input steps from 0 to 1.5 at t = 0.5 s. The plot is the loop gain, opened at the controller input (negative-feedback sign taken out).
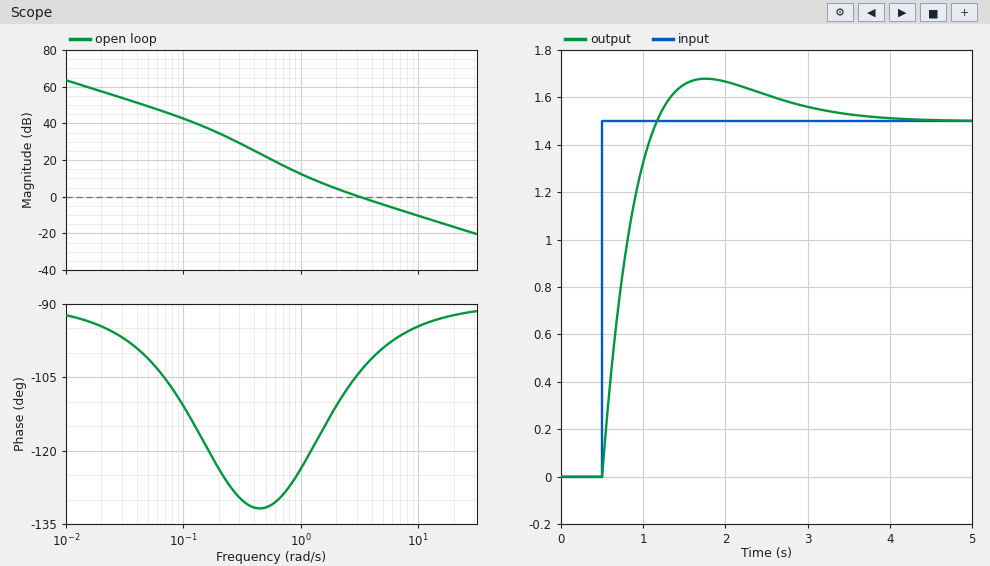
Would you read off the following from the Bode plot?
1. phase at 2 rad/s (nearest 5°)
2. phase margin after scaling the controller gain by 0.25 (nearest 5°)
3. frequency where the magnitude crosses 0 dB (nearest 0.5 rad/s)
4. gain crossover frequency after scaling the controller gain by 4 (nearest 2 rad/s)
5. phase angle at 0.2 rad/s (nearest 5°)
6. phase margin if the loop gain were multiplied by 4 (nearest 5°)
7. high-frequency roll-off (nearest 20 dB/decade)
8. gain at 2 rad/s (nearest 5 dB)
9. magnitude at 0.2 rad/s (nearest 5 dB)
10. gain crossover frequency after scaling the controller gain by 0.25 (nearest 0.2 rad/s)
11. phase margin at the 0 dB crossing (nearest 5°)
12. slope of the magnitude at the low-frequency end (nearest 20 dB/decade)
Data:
-110°
55°
3.0 rad/s
12 rad/s
-125°
85°
-20 dB/decade
5 dB
35 dB
1.0 rad/s
75°
-20 dB/decade
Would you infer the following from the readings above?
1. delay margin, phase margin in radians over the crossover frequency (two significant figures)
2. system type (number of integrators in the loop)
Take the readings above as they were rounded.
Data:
0.44 s
1
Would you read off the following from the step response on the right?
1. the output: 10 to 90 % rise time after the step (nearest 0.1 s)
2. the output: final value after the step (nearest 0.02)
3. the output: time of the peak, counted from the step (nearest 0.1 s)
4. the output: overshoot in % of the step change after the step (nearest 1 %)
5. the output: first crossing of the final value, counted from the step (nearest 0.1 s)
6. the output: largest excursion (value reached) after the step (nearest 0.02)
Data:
0.5 s
1.50
1.3 s
12 %
0.7 s
1.68
